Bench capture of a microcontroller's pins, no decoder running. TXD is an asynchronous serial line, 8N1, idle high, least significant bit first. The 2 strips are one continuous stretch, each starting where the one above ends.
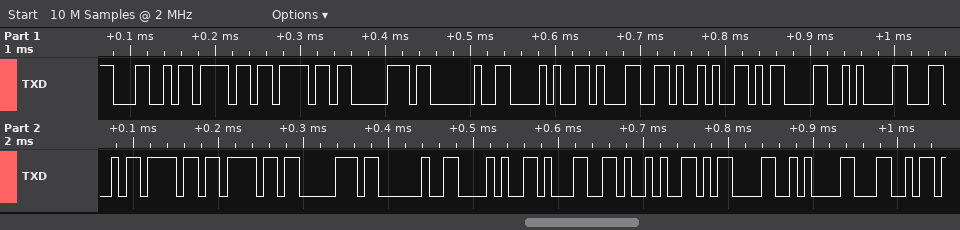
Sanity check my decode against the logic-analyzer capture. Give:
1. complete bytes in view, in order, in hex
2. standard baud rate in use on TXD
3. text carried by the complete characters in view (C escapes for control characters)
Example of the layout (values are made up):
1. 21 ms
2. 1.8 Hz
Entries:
1. 4C 6F 6F 70 20 28 31 29 0D 0A 4C 6F 6F 70 20 28 31 29 0D 0A 4C
2. 115200 baud
3. "Loop (1)\r\nLoop (1)\r\nL"
